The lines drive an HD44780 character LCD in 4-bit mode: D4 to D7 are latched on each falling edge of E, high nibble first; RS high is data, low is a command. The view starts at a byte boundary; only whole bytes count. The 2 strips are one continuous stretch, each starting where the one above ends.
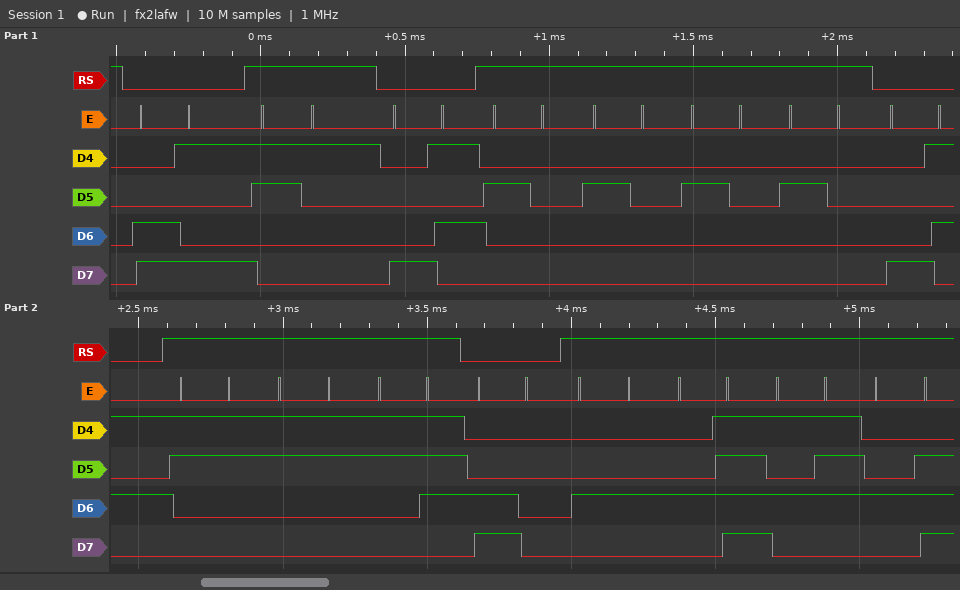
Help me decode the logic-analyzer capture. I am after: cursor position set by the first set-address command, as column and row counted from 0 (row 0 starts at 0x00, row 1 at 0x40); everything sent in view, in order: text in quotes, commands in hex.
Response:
column 9, row 1
0xC9 "1" 0x85 "    " 0x85 "337" 0xC0 "DOWN"
